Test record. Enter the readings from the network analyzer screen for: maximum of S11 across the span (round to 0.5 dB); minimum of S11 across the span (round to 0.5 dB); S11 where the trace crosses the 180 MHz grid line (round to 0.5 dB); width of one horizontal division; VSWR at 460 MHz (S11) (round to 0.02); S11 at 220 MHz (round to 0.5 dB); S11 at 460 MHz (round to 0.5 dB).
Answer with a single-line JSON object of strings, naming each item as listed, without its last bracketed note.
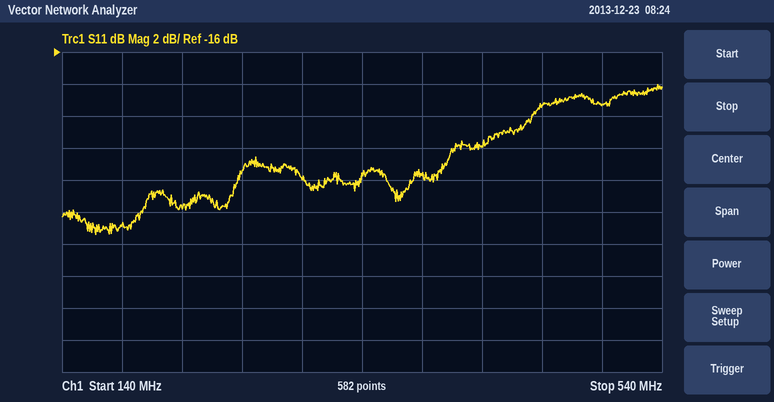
{"maximum of S11 across the span": "-18.0 dB", "minimum of S11 across the span": "-27.5 dB", "S11 where the trace crosses the 180 MHz grid line": "-27.0 dB", "width of one horizontal division": "40 MHz", "VSWR at 460 MHz (S11)": "1.24", "S11 at 220 MHz": "-25.5 dB", "S11 at 460 MHz": "-19.5 dB"}
